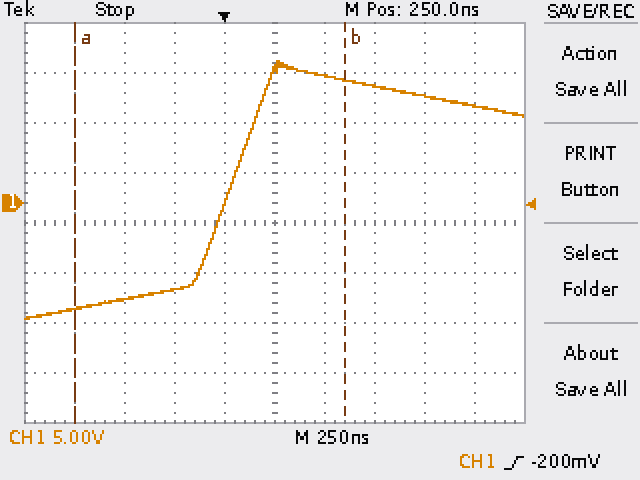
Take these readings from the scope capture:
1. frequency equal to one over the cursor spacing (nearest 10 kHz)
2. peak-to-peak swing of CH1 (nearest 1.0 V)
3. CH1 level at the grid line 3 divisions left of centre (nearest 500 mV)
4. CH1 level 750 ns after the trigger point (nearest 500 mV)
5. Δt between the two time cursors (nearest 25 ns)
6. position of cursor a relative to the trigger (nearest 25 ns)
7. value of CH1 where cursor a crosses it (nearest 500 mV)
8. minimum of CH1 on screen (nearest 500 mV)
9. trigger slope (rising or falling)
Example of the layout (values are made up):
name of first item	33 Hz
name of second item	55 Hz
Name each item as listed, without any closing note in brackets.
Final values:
frequency equal to one over the cursor spacing	740 kHz
peak-to-peak swing of CH1	26.0 V
CH1 level at the grid line 3 divisions left of centre	-9.5 V
CH1 level 750 ns after the trigger point	11.5 V
Δt between the two time cursors	1.350 µs
position of cursor a relative to the trigger	-750 ns
value of CH1 where cursor a crosses it	-10.5 V
minimum of CH1 on screen	-11.5 V
trigger slope	rising
